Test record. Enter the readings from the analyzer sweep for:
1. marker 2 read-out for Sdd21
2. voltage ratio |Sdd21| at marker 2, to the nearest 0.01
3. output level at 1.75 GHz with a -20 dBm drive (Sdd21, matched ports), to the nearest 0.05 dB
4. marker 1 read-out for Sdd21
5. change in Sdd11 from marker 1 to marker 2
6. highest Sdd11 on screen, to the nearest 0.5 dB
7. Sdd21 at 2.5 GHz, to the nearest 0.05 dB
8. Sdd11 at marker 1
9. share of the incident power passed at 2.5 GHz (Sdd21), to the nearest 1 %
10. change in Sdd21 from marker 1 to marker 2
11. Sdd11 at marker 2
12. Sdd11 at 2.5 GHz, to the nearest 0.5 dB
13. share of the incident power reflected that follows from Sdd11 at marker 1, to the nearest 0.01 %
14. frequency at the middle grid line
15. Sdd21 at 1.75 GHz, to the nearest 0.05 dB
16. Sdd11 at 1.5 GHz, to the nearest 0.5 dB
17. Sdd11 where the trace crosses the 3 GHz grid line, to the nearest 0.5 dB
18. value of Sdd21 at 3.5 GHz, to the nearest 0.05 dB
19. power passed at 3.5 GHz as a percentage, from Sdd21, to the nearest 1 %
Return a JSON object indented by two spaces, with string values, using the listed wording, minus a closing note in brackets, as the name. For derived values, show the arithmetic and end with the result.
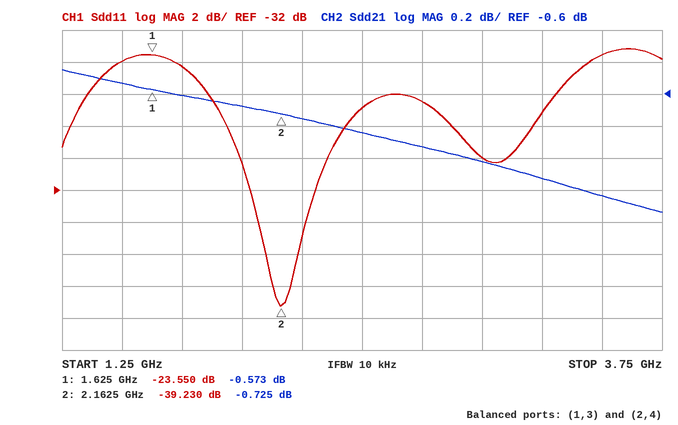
{
  "marker 2 read-out for Sdd21": "-0.725 dB",
  "voltage ratio |Sdd21| at marker 2, to the nearest 0.01": "10^(-0.725/20) ≈ 0.92",
  "output level at 1.75 GHz with a -20 dBm drive (Sdd21, matched ports), to the nearest 0.05 dB": "-20 dBm + (-0.60 dB) = -20.60 dBm",
  "marker 1 read-out for Sdd21": "-0.573 dB",
  "change in Sdd11 from marker 1 to marker 2": "-39.23 − (-23.55) = -15.680 dB",
  "highest Sdd11 on screen, to the nearest 0.5 dB": "-23.0 dB",
  "Sdd21 at 2.5 GHz, to the nearest 0.05 dB": "-0.85 dB",
  "Sdd11 at marker 1": "-23.550 dB",
  "share of the incident power passed at 2.5 GHz (Sdd21), to the nearest 1 %": "10^(-0.85/10) ≈ 82 %",
  "change in Sdd21 from marker 1 to marker 2": "-0.725 − (-0.573) = -0.152 dB",
  "Sdd11 at marker 2": "-39.230 dB",
  "Sdd11 at 2.5 GHz, to the nearest 0.5 dB": "-27.0 dB",
  "share of the incident power reflected that follows from Sdd11 at marker 1, to the nearest 0.01 %": "10^(-23.55/10) ≈ 0.44 %",
  "frequency at the middle grid line": "2.5 GHz",
  "Sdd21 at 1.75 GHz, to the nearest 0.05 dB": "-0.60 dB",
  "Sdd11 at 1.5 GHz, to the nearest 0.5 dB": "-24.0 dB",
  "Sdd11 where the trace crosses the 3 GHz grid line, to the nearest 0.5 dB": "-30.0 dB",
  "value of Sdd21 at 3.5 GHz, to the nearest 0.05 dB": "-1.25 dB",
  "power passed at 3.5 GHz as a percentage, from Sdd21, to the nearest 1 %": "10^(-1.25/10) ≈ 75 %"
}
